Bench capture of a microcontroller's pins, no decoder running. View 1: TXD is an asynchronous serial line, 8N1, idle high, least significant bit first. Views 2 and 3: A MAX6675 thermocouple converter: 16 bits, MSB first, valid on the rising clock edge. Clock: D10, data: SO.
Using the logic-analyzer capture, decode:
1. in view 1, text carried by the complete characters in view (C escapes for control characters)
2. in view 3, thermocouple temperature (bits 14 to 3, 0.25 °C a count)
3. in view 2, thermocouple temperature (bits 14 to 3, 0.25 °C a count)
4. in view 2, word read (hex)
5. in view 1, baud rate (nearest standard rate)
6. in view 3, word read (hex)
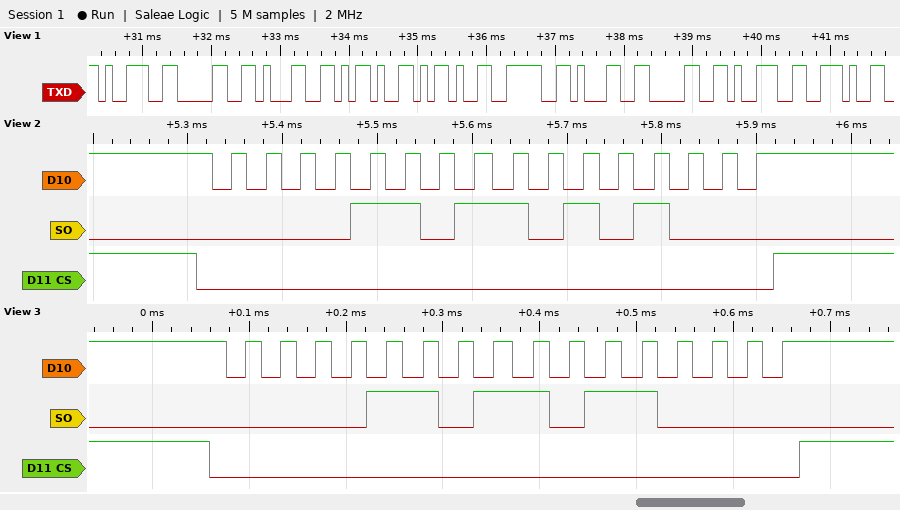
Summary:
"901-->109."
109.50 °C
109.25 °C
0x0DA8
9600 baud
0x0DB0
